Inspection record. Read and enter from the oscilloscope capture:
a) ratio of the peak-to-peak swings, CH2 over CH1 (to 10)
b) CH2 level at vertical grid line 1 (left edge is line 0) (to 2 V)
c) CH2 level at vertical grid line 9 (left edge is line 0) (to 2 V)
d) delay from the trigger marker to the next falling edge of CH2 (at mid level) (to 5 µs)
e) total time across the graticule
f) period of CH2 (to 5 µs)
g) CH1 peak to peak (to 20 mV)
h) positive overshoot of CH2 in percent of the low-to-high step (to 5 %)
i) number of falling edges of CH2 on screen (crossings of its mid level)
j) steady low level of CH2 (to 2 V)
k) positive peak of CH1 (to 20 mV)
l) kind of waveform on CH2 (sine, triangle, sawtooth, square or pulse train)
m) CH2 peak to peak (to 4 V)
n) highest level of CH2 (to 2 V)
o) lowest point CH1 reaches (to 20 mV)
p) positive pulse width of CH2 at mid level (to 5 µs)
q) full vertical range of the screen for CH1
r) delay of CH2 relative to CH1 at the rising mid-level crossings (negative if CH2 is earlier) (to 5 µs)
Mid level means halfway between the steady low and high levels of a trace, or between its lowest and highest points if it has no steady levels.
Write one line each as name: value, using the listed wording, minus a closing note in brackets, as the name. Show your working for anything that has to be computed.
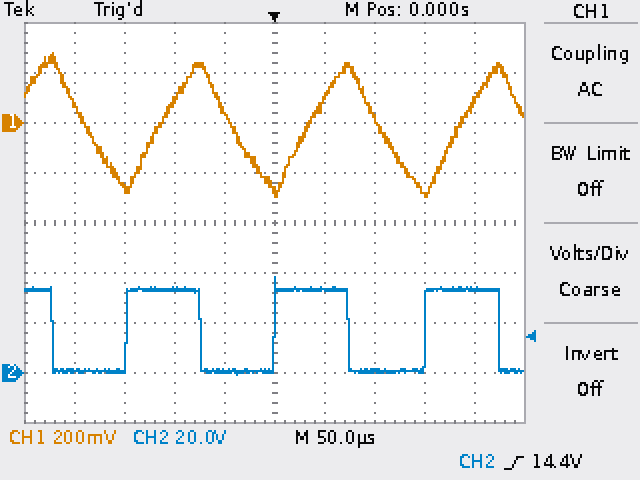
ratio of the peak-to-peak swings, CH2 over CH1: 40 V / 580 mV ≈ 69.0, so 70 to the nearest 10
CH2 level at vertical grid line 1 (left edge is line 0): 0 V
CH2 level at vertical grid line 9 (left edge is line 0): 34 V
delay from the trigger marker to the next falling edge of CH2 (at mid level): 75 µs
total time across the graticule: 500 µs
period of CH2: 150 µs
CH1 peak to peak: 280 mV − (-300 mV) = 580 mV
positive overshoot of CH2 in percent of the low-to-high step: 15 %
number of falling edges of CH2 on screen: 4
steady low level of CH2: 0 V
positive peak of CH1: 280 mV
kind of waveform on CH2: square
CH2 peak to peak: 40 V
highest level of CH2: 38 V
lowest point CH1 reaches: -300 mV
positive pulse width of CH2 at mid level: 75 µs
full vertical range of the screen for CH1: 1.6 V
delay of CH2 relative to CH1 at the rising mid-level crossings (negative if CH2 is earlier): -35 µs
